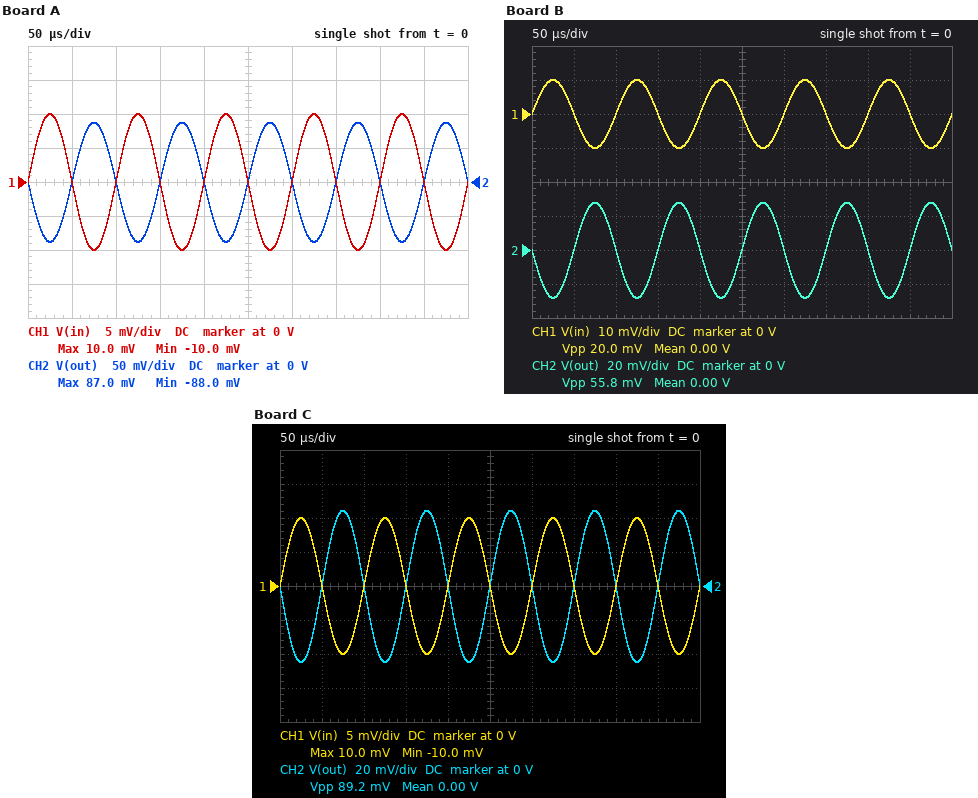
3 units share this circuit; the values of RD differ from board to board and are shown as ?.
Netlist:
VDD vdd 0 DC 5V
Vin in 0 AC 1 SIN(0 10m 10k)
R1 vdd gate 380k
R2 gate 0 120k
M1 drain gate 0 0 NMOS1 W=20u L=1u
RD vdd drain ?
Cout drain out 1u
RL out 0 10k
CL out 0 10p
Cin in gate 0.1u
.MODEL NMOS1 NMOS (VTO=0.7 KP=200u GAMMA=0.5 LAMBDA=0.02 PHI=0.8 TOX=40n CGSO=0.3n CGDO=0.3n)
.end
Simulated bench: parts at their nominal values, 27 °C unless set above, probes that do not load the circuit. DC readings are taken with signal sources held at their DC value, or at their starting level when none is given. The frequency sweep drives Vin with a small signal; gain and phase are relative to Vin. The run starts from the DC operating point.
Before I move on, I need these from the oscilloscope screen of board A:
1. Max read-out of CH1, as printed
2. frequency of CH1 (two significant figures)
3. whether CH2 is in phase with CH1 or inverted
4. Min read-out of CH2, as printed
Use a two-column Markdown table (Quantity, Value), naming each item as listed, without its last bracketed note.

| Quantity | Value |
|---|---|
| Max read-out of CH1, as printed | 10.0 mV |
| frequency of CH1 | 10 kHz |
| whether CH2 is in phase with CH1 or inverted | inverted |
| Min read-out of CH2, as printed | -88.0 mV |
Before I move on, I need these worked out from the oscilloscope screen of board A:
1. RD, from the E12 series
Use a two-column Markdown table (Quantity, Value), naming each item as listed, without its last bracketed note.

| Quantity | Value |
|---|---|
| RD, from the E12 series | 8.2 kΩ |
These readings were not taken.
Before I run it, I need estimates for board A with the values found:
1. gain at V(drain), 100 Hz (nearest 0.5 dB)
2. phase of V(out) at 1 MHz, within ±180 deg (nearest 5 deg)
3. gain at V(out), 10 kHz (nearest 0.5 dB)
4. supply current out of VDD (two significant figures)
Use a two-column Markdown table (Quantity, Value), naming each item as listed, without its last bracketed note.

| Quantity | Value |
|---|---|
| gain at V(drain), 100 Hz | 19.0 dB |
| phase of V(out) at 1 MHz, within ±180 deg | 165 deg |
| gain at V(out), 10 kHz | 19.0 dB |
| supply current out of VDD | 520 µA |
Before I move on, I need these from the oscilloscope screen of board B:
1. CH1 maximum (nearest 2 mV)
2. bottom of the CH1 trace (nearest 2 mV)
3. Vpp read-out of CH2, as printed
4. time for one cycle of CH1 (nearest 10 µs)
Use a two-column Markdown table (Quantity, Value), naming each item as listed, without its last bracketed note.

| Quantity | Value |
|---|---|
| CH1 maximum | 10 mV |
| bottom of the CH1 trace | -10 mV |
| Vpp read-out of CH2, as printed | 55.8 mV |
| time for one cycle of CH1 | 100 µs |
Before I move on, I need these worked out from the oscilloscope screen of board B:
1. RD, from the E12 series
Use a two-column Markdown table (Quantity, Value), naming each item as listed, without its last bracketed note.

| Quantity | Value |
|---|---|
| RD, from the E12 series | 1.5 kΩ |
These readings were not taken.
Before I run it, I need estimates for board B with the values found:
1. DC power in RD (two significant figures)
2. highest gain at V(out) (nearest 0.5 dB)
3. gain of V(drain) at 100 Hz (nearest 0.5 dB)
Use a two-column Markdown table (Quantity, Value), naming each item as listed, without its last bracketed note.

| Quantity | Value |
|---|---|
| DC power in RD | 440 µW |
| highest gain at V(out) | 9.0 dB |
| gain of V(drain) at 100 Hz | 9.0 dB |
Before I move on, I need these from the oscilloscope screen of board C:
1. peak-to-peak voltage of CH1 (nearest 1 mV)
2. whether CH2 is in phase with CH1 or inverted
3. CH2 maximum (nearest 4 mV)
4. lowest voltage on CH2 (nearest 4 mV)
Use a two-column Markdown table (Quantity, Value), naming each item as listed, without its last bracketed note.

| Quantity | Value |
|---|---|
| peak-to-peak voltage of CH1 | 20 mV |
| whether CH2 is in phase with CH1 or inverted | inverted |
| CH2 maximum | 44 mV |
| lowest voltage on CH2 | -44 mV |
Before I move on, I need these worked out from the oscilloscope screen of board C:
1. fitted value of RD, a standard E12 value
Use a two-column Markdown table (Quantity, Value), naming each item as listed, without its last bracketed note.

| Quantity | Value |
|---|---|
| fitted value of RD, a standard E12 value | 2.7 kΩ |
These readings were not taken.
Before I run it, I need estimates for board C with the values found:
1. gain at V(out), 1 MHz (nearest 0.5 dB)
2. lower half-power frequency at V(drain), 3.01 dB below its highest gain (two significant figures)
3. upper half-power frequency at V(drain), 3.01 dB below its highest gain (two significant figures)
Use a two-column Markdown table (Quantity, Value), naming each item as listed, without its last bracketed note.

| Quantity | Value |
|---|---|
| gain at V(out), 1 MHz | 13.0 dB |
| lower half-power frequency at V(drain), 3.01 dB below its highest gain | 14 Hz |
| upper half-power frequency at V(drain), 3.01 dB below its highest gain | 7.6 MHz |
